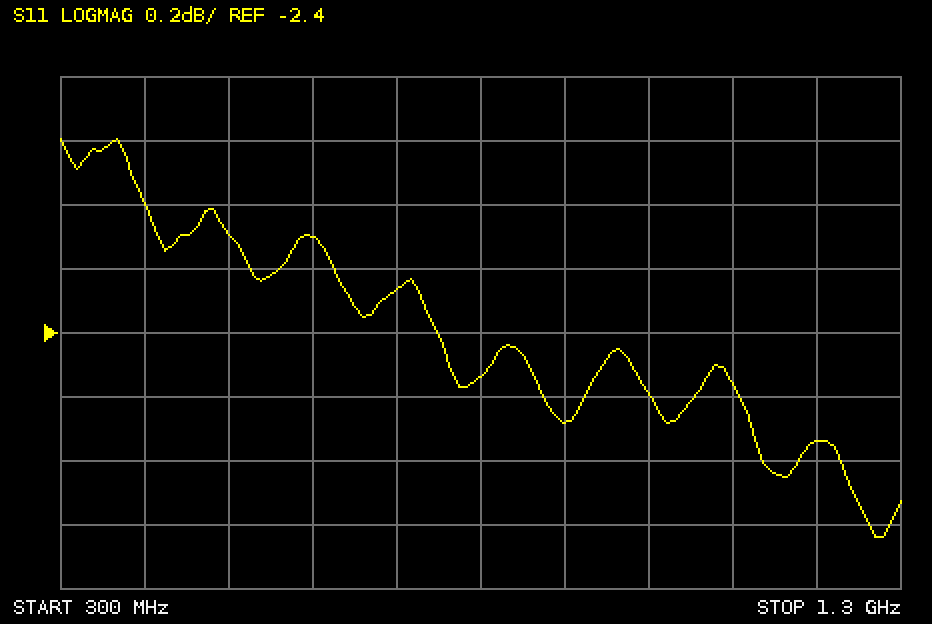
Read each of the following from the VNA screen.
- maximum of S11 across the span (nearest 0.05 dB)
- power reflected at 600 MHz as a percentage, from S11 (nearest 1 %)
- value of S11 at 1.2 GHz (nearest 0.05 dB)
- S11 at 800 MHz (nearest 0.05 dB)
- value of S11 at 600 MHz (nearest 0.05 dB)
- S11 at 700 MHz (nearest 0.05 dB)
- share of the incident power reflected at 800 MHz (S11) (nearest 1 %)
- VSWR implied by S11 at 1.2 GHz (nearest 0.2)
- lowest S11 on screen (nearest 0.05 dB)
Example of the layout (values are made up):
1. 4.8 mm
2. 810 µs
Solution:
1. -1.80 dB
2. 62 %
3. -2.75 dB
4. -2.55 dB
5. -2.10 dB
6. -2.25 dB
7. 56 %
8. 6.4
9. -3.05 dB
